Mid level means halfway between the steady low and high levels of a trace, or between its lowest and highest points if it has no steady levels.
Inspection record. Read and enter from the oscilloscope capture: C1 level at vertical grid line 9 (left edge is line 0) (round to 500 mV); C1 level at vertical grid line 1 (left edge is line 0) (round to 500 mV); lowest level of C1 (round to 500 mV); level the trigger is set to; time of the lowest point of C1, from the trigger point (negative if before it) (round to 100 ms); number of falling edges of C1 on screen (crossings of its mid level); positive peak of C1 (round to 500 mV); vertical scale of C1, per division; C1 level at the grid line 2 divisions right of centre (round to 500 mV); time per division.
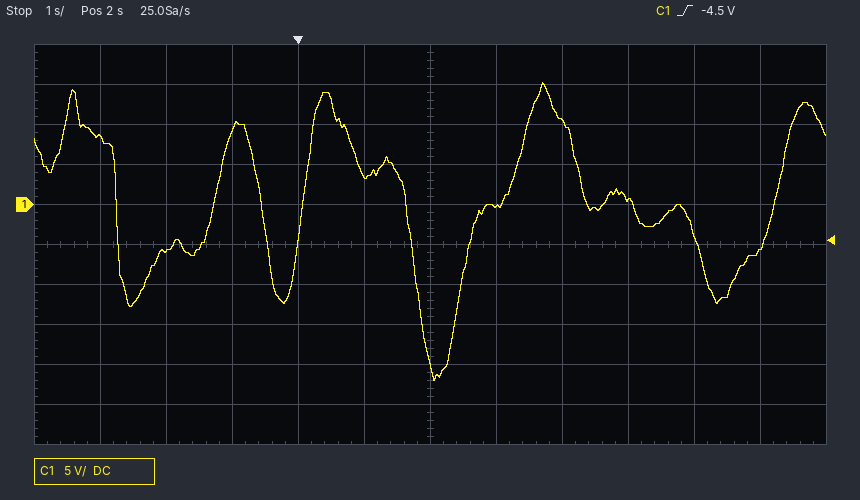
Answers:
500 mV
8.5 V
-22.0 V
-4.5 V
+2.1 s
4
15.0 V
5 V
10.5 V
1 s
